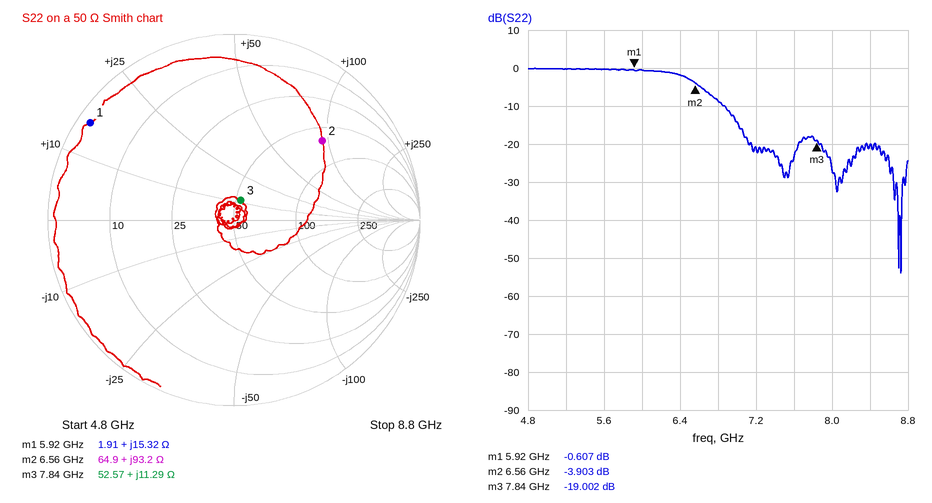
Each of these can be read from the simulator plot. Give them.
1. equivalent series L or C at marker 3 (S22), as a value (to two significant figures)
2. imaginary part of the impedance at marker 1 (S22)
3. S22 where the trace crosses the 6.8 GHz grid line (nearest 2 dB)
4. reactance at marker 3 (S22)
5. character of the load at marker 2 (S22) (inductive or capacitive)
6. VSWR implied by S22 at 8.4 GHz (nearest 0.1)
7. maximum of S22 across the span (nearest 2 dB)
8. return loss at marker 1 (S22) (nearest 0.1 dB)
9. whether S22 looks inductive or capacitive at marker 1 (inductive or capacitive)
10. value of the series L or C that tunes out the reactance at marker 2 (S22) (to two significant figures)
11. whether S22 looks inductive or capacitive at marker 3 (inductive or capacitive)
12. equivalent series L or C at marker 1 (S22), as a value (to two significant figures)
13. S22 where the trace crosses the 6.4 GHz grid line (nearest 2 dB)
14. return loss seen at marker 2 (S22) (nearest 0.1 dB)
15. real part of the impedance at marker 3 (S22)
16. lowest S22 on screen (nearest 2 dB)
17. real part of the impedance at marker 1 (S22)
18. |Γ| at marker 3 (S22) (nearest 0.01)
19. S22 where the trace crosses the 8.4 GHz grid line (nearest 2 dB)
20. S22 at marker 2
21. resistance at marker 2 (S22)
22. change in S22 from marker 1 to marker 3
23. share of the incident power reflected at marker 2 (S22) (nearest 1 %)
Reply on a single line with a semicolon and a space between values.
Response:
230 pH; +15.32 Ω; -8 dB; +11.29 Ω; inductive; 1.2; 0 dB; 0.6 dB; inductive; 260 fF; inductive; 410 pH; -2 dB; 3.9 dB; 52.57 Ω; -54 dB; 1.91 Ω; 0.11; -20 dB; -3.903 dB; 64.9 Ω; -18.395 dB; 41 %
